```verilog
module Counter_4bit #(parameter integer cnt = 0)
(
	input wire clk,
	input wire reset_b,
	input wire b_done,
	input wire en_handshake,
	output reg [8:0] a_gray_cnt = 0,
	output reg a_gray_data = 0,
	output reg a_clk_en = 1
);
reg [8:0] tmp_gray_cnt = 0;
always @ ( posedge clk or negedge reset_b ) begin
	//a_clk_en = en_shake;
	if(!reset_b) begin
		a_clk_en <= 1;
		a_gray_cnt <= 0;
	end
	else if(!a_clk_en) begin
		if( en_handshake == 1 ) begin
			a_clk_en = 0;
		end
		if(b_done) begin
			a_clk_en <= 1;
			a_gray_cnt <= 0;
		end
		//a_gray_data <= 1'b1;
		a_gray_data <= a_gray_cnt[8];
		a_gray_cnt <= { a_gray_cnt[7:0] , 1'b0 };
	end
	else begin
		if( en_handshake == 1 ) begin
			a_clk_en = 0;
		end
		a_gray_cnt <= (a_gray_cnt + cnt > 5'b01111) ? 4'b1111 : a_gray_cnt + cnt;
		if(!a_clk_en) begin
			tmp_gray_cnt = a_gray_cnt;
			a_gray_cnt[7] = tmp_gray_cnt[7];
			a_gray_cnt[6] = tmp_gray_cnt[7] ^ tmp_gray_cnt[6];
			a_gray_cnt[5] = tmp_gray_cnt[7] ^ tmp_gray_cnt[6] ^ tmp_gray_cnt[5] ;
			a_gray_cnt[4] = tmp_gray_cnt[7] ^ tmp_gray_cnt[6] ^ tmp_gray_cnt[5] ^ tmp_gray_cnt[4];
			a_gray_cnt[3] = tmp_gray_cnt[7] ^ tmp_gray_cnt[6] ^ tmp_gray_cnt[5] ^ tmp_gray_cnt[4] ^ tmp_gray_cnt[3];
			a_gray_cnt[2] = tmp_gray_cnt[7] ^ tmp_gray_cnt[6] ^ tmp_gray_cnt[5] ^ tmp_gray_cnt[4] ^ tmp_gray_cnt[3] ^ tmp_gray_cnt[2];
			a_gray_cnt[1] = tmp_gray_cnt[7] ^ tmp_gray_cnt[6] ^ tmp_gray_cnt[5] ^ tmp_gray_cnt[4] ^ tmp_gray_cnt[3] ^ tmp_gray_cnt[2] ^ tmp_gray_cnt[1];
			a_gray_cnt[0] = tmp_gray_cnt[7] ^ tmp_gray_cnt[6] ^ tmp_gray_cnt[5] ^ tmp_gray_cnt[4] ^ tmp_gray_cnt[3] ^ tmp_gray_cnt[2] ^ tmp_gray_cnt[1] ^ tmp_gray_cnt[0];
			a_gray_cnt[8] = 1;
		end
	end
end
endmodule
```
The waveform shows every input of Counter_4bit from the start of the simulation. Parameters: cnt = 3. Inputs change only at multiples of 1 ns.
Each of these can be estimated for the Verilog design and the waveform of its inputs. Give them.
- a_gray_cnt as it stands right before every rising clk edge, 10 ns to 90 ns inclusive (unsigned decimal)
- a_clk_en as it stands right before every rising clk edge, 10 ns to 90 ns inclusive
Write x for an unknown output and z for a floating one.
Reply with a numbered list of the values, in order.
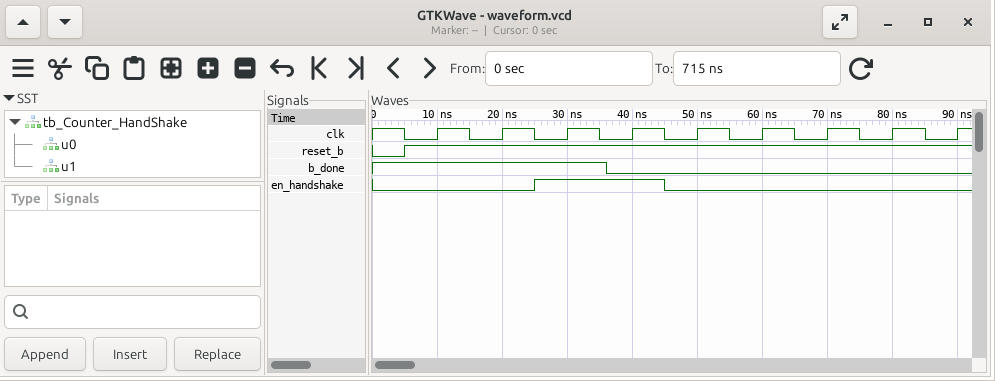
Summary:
1. 0, 3, 6, 9, 18, 36, 72, 144, 288
2. 1 1 1 0 0 0 0 0 0
